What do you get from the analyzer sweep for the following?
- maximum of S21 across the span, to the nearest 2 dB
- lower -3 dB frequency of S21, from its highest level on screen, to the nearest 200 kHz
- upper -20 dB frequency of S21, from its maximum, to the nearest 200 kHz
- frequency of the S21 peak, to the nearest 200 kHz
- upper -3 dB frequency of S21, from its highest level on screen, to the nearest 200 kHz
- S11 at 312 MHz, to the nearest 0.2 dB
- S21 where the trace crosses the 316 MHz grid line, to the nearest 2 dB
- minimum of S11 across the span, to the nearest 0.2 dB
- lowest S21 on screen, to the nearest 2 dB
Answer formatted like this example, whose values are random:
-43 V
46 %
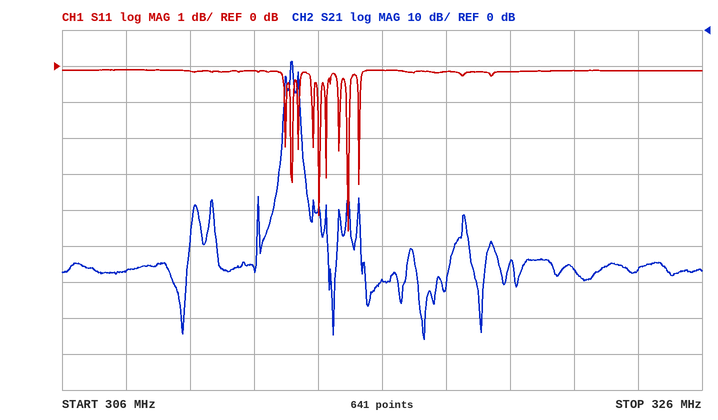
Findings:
-8 dB
313.2 MHz
313.4 MHz
313.2 MHz
313.2 MHz
-0.2 dB
-70 dB
-4.6 dB
-86 dB
